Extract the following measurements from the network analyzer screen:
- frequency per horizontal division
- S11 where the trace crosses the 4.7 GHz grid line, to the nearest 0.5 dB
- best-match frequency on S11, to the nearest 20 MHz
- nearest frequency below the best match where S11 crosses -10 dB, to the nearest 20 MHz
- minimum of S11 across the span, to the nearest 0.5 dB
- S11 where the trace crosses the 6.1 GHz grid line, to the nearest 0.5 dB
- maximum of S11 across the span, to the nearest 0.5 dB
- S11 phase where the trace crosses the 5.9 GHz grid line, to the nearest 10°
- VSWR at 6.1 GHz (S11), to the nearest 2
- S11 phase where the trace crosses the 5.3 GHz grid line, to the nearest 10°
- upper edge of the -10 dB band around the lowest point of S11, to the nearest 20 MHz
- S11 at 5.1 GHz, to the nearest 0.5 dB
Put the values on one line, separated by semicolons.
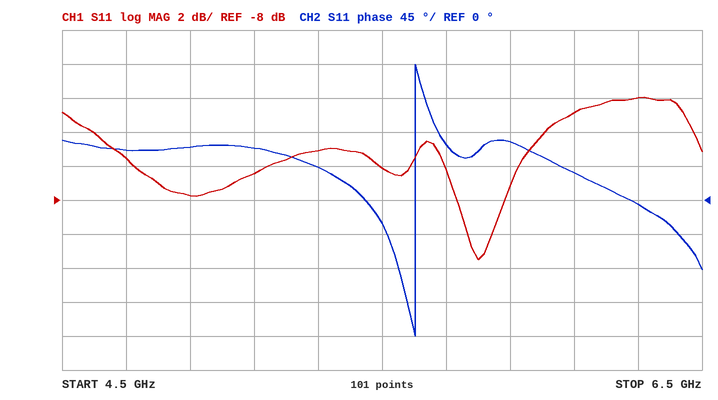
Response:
200 MHz; -5.5 dB; 5.80 GHz; 5.76 GHz; -11.5 dB; -3.0 dB; -2.0 dB; 80°; 6; 40°; 5.84 GHz; -6.5 dB
